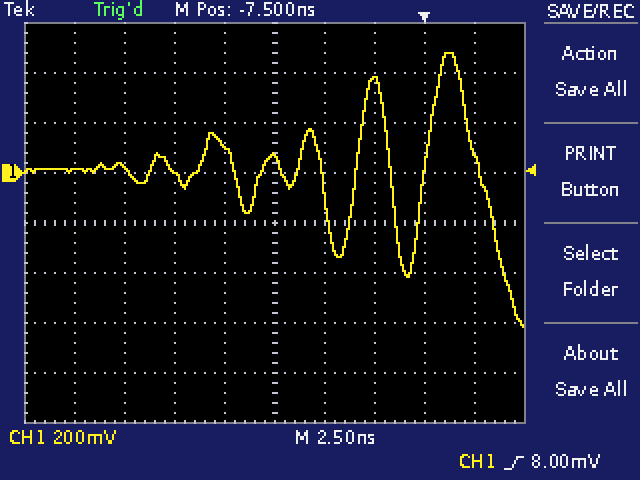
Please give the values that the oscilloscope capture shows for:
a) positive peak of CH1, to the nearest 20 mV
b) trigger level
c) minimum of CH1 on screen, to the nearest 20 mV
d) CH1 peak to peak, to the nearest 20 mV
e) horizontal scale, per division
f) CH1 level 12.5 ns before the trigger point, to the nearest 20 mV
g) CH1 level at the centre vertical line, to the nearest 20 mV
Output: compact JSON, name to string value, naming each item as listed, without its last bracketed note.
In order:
{"positive peak of CH1, to the nearest 20 mV": "480 mV", "trigger level": "8.00 mV", "minimum of CH1 on screen, to the nearest 20 mV": "-620 mV", "CH1 peak to peak, to the nearest 20 mV": "1.10 V", "horizontal scale, per division": "2.5 ns", "CH1 level 12.5 ns before the trigger point, to the nearest 20 mV": "0 mV", "CH1 level at the centre vertical line, to the nearest 20 mV": "60 mV"}
